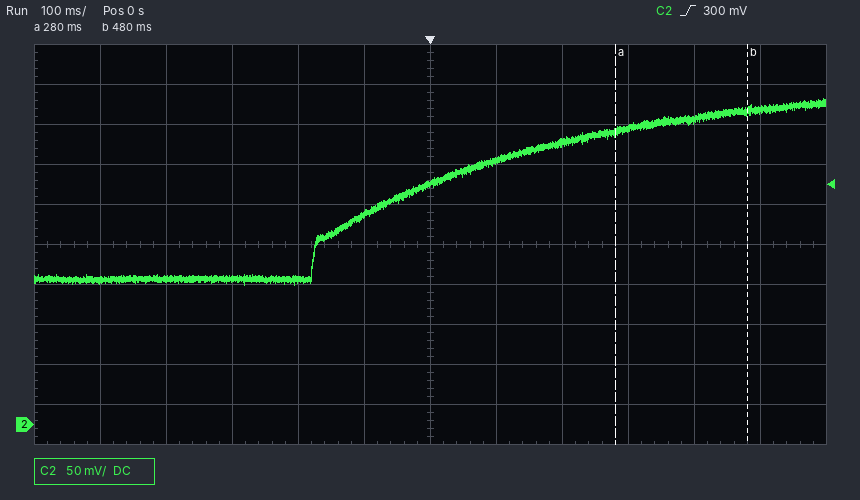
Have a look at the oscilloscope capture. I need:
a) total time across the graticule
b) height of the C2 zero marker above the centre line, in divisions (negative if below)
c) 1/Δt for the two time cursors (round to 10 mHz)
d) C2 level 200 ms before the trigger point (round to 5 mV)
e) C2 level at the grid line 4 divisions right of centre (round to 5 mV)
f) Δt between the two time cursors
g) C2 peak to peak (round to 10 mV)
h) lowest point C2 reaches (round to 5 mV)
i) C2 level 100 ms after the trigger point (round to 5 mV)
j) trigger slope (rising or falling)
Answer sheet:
1.2 s
-4.5 div
5.00 Hz
180 mV
380 mV
200 ms
230 mV
175 mV
330 mV
rising
